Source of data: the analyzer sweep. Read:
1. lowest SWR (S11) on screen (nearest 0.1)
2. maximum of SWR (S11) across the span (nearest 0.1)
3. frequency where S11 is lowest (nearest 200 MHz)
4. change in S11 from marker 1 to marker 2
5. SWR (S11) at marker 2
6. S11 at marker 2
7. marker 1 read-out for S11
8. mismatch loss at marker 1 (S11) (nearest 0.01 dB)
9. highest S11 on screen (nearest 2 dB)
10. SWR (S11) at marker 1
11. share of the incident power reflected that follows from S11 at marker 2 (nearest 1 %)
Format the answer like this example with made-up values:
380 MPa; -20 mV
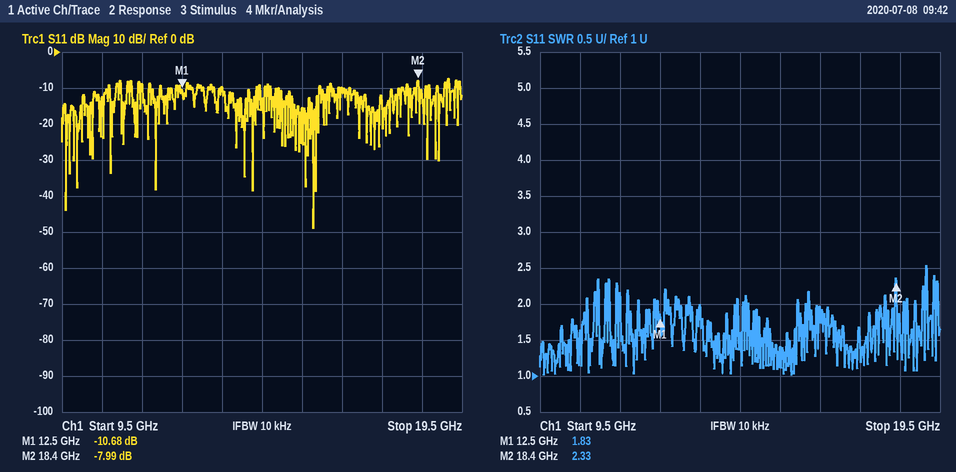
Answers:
1.0; 2.5; 15.8 GHz; 2.69 dB; 2.33; -7.99 dB; -10.68 dB; 0.39 dB; -8 dB; 1.83; 16 %
